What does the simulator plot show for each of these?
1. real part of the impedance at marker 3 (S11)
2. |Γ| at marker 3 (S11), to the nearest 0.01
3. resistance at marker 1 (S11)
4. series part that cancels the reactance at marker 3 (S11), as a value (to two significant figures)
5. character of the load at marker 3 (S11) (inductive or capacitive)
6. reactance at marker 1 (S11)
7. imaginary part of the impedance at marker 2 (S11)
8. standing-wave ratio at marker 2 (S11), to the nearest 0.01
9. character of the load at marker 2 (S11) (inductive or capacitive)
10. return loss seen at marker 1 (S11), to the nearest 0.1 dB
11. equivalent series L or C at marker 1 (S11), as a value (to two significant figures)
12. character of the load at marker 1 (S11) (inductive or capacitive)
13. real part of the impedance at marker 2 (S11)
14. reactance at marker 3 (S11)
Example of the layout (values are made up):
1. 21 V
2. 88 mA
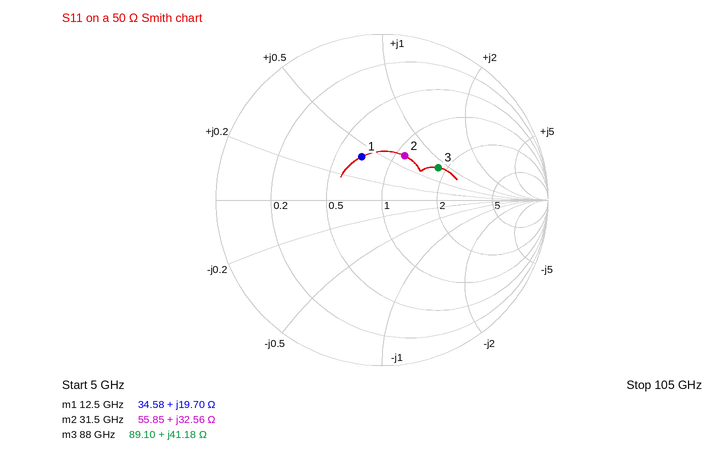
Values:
1. 89.10 Ω
2. 0.39
3. 34.58 Ω
4. 44 fF
5. inductive
6. +19.70 Ω
7. +32.56 Ω
8. 1.85
9. inductive
10. 10.8 dB
11. 250 pH
12. inductive
13. 55.85 Ω
14. +41.18 Ω
